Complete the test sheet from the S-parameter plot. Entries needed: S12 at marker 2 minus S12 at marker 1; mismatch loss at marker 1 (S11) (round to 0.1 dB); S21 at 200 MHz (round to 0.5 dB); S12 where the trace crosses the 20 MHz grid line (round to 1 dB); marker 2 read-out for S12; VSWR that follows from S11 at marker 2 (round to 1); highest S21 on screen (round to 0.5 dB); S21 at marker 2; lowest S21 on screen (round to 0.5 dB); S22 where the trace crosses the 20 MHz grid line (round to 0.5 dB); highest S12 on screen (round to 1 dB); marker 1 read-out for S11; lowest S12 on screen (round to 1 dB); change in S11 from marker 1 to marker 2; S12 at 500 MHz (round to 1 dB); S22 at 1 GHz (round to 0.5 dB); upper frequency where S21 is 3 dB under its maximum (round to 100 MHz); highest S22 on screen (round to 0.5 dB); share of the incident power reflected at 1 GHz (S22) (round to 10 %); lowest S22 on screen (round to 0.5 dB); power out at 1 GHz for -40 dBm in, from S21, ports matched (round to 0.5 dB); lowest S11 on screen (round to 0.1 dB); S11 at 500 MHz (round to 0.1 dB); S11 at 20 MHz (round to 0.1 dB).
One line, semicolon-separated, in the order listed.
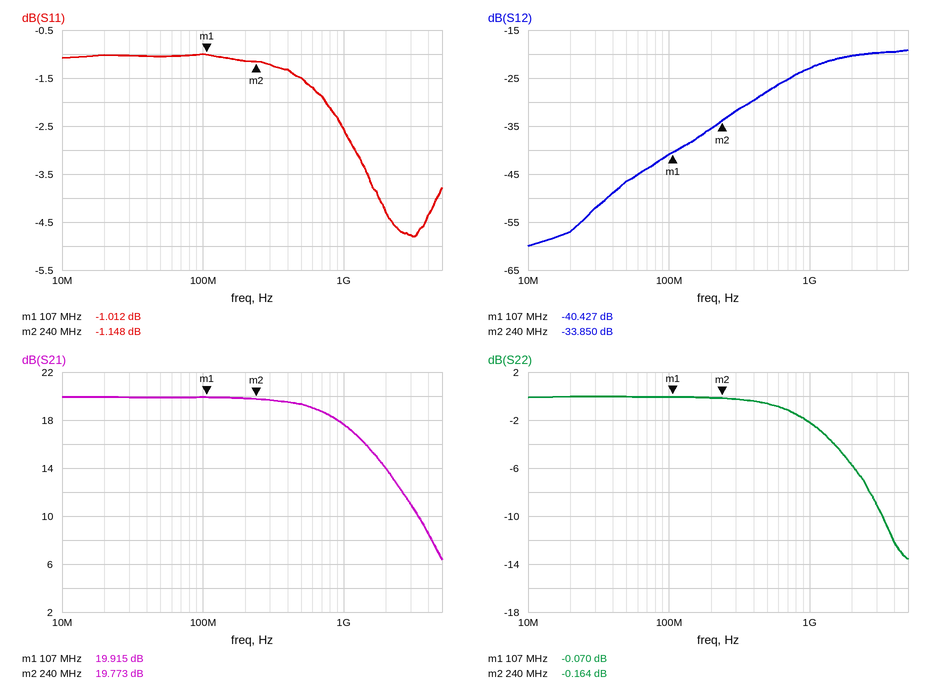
6.577 dB; 6.8 dB; 20.0 dB; -57 dB; -33.850 dB; 15; 20.0 dB; 19.773 dB; 6.5 dB; 0.0 dB; -19 dB; -1.012 dB; -60 dB; -0.136 dB; -28 dB; -2.0 dB; 1.2 GHz; 0.0 dB; 60 %; -13.5 dB; -22.5 dBm; -4.8 dB; -1.5 dB; -1.0 dB
